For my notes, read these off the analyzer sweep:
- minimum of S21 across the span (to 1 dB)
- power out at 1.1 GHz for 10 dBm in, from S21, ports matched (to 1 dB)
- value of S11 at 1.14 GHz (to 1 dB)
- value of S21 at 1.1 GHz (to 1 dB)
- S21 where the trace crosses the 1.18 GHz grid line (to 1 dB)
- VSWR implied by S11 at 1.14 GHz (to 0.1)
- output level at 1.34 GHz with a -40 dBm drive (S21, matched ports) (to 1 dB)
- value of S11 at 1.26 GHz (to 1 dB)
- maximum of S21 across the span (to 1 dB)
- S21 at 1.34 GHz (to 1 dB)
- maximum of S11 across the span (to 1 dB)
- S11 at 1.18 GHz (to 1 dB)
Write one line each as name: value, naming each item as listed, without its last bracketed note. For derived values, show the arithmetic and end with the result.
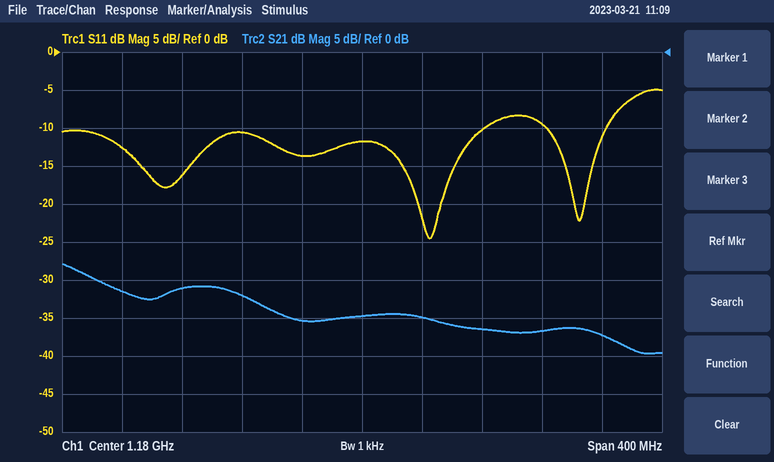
minimum of S21 across the span: -40 dB
power out at 1.1 GHz for 10 dBm in, from S21, ports matched: 10 dBm + (-32 dB) = -22 dBm
value of S11 at 1.14 GHz: -14 dB
value of S21 at 1.1 GHz: -32 dB
S21 where the trace crosses the 1.18 GHz grid line: -35 dB
VSWR implied by S11 at 1.14 GHz: |Γ| = 10^(-14/20) = 0.1995; VSWR = (1 + 0.1995)/(1 − 0.1995) ≈ 1.5
output level at 1.34 GHz with a -40 dBm drive (S21, matched ports): -40 dBm + (-37 dB) = -77 dBm
value of S11 at 1.26 GHz: -10 dB
maximum of S21 across the span: -28 dB
S21 at 1.34 GHz: -37 dB
maximum of S11 across the span: -5 dB
S11 at 1.18 GHz: -12 dB
